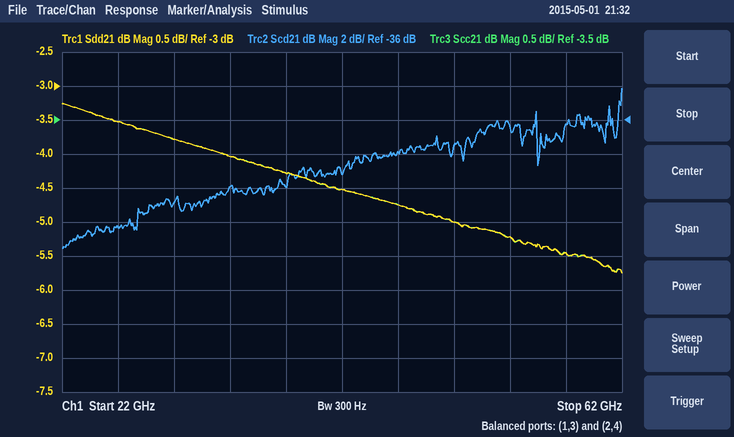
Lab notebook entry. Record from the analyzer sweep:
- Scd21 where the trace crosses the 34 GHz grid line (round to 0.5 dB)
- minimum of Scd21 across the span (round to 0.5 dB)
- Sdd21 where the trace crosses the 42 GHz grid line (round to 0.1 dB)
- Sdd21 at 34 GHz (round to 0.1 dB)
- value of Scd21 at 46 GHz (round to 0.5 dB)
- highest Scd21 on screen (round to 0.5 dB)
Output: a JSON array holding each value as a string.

["-40.0 dB", "-43.5 dB", "-4.5 dB", "-4.0 dB", "-38.0 dB", "-34.0 dB"]
